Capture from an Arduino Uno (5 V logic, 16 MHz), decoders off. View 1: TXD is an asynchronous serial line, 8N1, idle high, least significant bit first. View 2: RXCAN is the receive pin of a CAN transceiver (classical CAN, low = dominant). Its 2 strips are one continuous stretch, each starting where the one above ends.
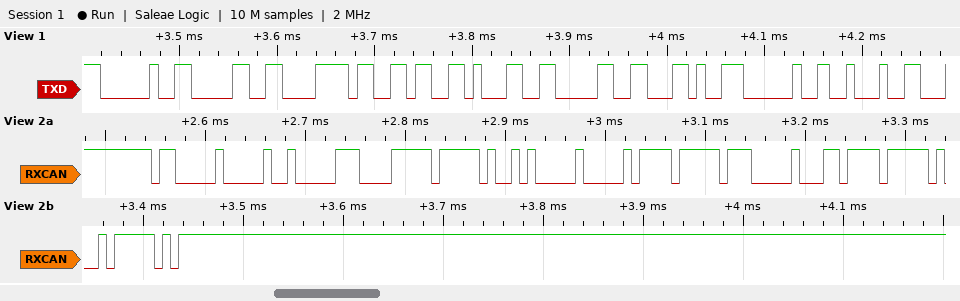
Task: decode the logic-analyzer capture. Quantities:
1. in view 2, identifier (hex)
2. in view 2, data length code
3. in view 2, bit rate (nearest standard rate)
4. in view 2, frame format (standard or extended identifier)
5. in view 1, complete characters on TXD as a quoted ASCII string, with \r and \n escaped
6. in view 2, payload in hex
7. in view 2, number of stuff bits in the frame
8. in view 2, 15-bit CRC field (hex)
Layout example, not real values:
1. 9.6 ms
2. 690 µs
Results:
1. 0x600
2. 8
3. 125 kbit/s
4. standard
5. " 0x610, \""
6. 30 FF E5 00 1E FF 00 DE
7. 11
8. 0x7E5F
